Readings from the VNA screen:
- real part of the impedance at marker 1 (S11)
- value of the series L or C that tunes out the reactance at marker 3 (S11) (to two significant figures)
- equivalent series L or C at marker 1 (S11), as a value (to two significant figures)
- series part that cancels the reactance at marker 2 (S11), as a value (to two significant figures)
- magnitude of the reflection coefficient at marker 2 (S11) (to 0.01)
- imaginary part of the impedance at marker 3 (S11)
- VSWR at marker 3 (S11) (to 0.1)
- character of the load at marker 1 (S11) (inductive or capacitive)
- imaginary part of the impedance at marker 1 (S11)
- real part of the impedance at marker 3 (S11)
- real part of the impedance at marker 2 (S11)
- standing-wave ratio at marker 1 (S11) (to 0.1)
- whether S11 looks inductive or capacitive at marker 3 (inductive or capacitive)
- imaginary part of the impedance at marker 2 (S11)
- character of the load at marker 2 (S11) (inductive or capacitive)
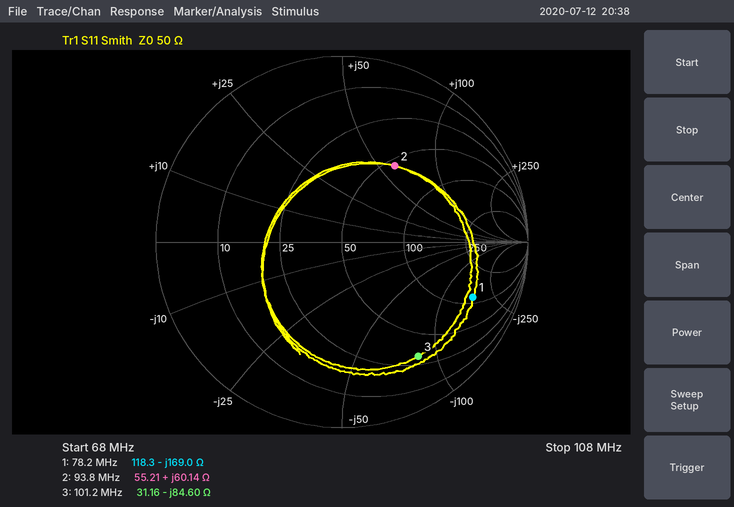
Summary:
118.3 Ω
130 nH
12 pF
28 pF
0.50
-84.60 Ω
6.7
capacitive
-169.0 Ω
31.16 Ω
55.21 Ω
7.5
capacitive
+60.14 Ω
inductive
